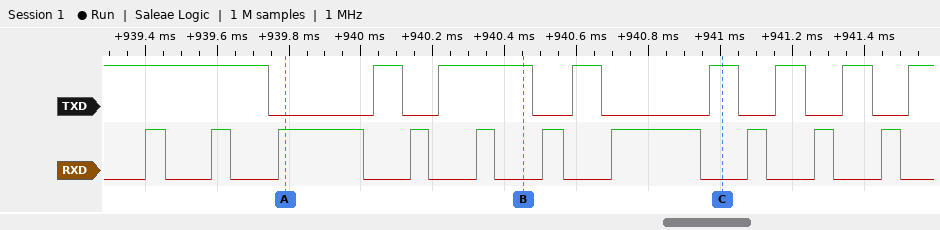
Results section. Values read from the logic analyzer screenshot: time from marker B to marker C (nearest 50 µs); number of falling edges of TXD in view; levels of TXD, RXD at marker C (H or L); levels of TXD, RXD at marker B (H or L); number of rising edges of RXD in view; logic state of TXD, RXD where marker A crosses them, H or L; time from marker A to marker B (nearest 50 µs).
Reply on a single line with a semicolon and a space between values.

550 µs; 7; TXD=H, RXD=L; TXD=H, RXD=L; 10; TXD=L, RXD=H; 650 µs
